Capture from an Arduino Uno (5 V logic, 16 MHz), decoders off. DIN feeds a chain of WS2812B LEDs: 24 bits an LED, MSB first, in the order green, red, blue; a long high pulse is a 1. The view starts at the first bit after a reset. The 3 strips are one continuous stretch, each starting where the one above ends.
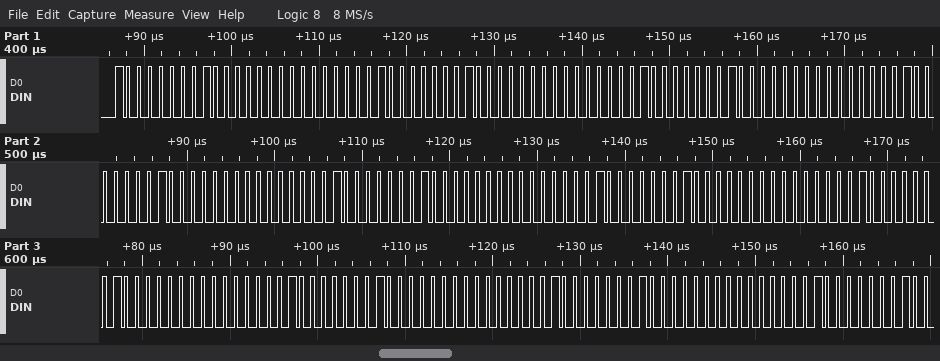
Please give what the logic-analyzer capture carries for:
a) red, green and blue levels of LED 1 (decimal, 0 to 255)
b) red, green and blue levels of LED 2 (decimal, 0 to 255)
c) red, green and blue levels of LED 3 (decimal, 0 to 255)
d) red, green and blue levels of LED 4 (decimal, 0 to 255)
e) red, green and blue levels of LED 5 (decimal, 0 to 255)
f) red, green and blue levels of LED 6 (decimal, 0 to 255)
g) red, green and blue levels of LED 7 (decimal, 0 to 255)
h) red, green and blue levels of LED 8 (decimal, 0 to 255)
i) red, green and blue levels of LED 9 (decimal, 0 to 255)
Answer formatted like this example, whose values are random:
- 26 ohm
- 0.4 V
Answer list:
- 128, 128, 0
- 128, 128, 0
- 128, 128, 0
- 128, 128, 0
- 128, 128, 0
- 128, 128, 0
- 128, 128, 0
- 128, 128, 0
- 128, 128, 0
